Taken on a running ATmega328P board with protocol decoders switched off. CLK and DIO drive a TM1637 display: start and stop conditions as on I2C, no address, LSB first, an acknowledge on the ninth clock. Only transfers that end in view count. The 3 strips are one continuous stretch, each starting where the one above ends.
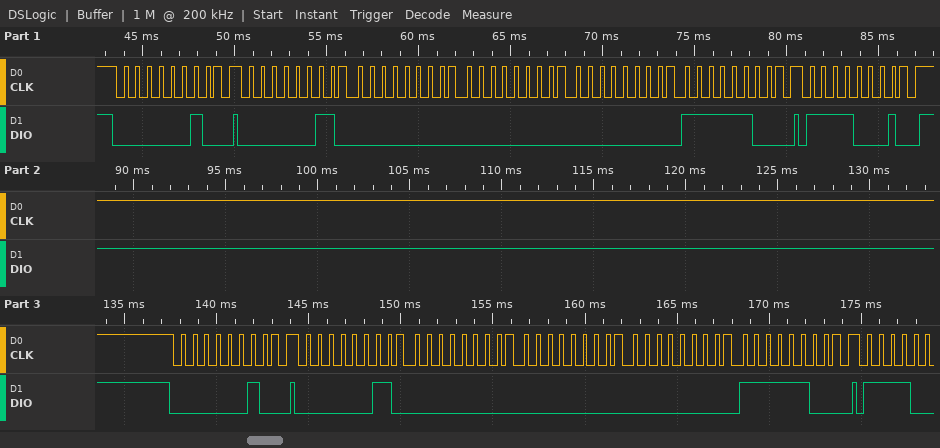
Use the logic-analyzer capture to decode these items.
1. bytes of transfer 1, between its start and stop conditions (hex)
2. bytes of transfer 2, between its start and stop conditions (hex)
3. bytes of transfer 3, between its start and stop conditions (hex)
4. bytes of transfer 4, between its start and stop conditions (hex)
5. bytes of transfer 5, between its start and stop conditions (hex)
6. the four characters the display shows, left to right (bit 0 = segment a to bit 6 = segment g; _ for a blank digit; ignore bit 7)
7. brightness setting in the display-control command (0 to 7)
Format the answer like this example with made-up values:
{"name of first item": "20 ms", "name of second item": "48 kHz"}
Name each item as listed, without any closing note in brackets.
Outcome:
{"bytes of transfer 1, between its start and stop conditions": "40", "bytes of transfer 2, between its start and stop conditions": "C0 00 00 00 3F", "bytes of transfer 3, between its start and stop conditions": "8F", "bytes of transfer 4, between its start and stop conditions": "40", "bytes of transfer 5, between its start and stop conditions": "C0 00 00 00 3F", "the four characters the display shows, left to right": "___0", "brightness setting in the display-control command": "7"}
